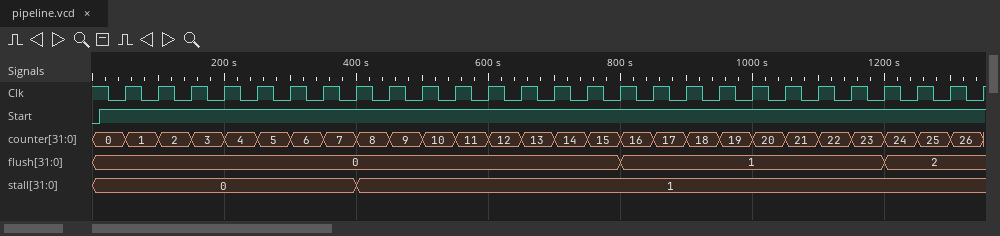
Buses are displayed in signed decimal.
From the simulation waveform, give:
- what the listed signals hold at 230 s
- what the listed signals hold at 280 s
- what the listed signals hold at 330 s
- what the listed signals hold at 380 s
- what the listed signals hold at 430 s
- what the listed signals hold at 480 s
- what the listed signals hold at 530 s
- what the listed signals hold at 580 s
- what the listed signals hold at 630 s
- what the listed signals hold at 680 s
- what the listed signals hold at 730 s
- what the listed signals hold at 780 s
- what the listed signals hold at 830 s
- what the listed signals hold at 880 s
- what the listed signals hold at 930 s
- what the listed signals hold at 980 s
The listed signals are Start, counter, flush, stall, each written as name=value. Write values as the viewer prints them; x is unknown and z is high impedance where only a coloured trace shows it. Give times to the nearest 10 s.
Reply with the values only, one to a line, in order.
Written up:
Start=1, counter=4, flush=0, stall=0
Start=1, counter=5, flush=0, stall=0
Start=1, counter=6, flush=0, stall=0
Start=1, counter=7, flush=0, stall=0
Start=1, counter=8, flush=0, stall=1
Start=1, counter=9, flush=0, stall=1
Start=1, counter=10, flush=0, stall=1
Start=1, counter=11, flush=0, stall=1
Start=1, counter=12, flush=0, stall=1
Start=1, counter=13, flush=0, stall=1
Start=1, counter=14, flush=0, stall=1
Start=1, counter=15, flush=0, stall=1
Start=1, counter=16, flush=1, stall=1
Start=1, counter=17, flush=1, stall=1
Start=1, counter=18, flush=1, stall=1
Start=1, counter=19, flush=1, stall=1
